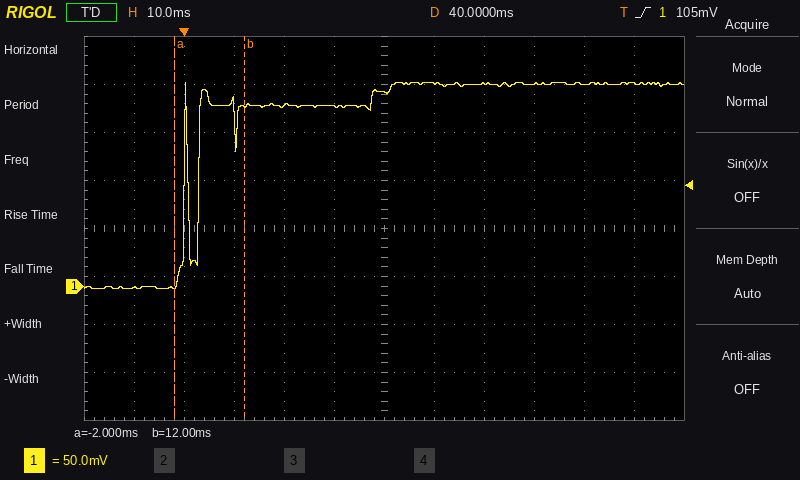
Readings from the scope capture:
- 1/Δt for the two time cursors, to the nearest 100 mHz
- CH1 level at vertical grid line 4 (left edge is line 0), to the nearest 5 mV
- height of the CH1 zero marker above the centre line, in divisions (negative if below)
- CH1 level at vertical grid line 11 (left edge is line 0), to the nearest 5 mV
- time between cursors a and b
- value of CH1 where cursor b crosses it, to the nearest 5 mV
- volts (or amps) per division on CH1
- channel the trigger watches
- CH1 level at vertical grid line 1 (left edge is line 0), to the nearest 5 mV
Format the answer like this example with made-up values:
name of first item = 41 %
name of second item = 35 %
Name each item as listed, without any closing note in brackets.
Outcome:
1/Δt for the two time cursors, to the nearest 100 mHz = 71.4 Hz
CH1 level at vertical grid line 4 (left edge is line 0), to the nearest 5 mV = 190 mV
height of the CH1 zero marker above the centre line, in divisions = -1.2 div
CH1 level at vertical grid line 11 (left edge is line 0), to the nearest 5 mV = 210 mV
time between cursors a and b = 14 ms
value of CH1 where cursor b crosses it, to the nearest 5 mV = 190 mV
volts (or amps) per division on CH1 = 50 mV
channel the trigger watches = CH1
CH1 level at vertical grid line 1 (left edge is line 0), to the nearest 5 mV = 0 mV
